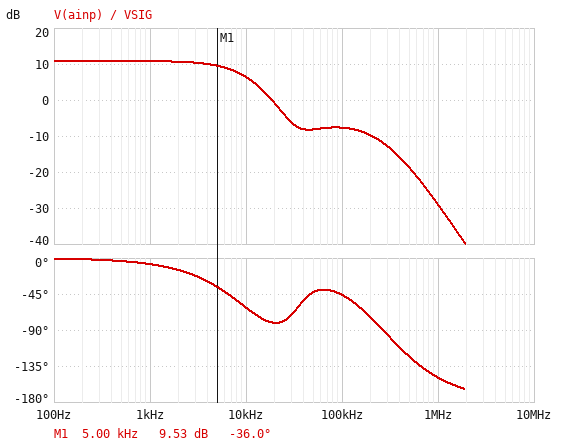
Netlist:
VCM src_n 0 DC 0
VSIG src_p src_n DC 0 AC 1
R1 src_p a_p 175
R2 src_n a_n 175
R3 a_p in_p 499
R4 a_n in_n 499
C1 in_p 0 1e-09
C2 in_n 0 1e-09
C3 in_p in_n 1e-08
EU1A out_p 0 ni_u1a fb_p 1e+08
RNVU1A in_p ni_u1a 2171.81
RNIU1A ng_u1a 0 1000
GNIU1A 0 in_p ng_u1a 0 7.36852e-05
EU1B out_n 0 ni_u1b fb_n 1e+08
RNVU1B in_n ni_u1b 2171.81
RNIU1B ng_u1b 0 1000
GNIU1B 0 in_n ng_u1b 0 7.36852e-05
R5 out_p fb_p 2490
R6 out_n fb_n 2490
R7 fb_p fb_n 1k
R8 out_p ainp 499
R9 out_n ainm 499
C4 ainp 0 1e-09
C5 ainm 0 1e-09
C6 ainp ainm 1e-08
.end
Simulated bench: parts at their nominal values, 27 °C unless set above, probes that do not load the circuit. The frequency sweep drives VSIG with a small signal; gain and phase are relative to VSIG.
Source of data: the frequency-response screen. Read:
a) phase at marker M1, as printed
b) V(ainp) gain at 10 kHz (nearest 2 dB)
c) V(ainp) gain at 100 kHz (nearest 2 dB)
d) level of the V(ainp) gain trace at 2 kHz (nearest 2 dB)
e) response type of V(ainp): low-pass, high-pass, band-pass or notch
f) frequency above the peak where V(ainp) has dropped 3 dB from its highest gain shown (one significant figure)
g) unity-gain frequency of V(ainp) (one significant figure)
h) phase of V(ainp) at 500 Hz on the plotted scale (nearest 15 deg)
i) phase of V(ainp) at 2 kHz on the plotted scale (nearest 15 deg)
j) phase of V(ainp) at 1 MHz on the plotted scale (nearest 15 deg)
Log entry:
-36.0 deg
6 dB
-8 dB
10 dB
low-pass
8 kHz
20 kHz
0 deg
-15 deg
-150 deg
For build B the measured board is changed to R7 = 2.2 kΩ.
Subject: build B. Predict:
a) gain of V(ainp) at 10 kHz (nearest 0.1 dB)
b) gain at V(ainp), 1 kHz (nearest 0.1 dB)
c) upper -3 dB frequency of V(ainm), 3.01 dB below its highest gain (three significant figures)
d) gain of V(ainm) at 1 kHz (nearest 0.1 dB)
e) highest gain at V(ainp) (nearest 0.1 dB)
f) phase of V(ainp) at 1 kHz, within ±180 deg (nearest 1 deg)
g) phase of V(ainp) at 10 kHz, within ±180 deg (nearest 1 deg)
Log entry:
2.1 dB
6.5 dB
18.6 kHz
1.1 dB
6.6 dB
-7 deg
-53 deg
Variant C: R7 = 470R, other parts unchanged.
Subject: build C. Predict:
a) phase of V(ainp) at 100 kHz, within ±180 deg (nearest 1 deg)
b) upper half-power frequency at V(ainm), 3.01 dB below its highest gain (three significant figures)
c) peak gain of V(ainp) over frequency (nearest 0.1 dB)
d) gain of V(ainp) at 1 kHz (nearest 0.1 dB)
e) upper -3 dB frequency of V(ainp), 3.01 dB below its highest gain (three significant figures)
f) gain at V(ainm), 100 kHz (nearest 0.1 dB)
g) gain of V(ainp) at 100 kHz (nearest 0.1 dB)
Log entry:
-52 deg
8.87 kHz
16.0 dB
15.9 dB
8.00 kHz
-6.0 dB
-8.1 dB
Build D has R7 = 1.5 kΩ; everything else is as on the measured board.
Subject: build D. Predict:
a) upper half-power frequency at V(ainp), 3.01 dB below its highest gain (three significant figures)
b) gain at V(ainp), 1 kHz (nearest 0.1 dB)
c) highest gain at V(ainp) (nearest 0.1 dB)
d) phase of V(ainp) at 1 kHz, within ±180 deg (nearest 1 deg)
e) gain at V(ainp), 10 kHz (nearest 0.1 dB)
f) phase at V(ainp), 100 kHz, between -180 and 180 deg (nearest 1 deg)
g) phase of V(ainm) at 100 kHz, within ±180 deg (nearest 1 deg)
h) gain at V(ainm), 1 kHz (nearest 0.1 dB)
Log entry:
7.85 kHz
8.4 dB
8.5 dB
-7 deg
4.0 dB
-44 deg
-37 deg
4.4 dB
